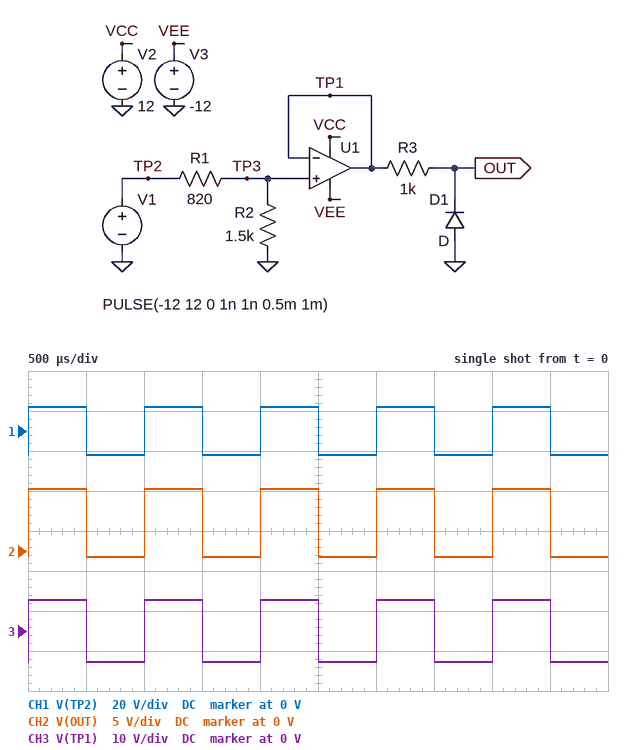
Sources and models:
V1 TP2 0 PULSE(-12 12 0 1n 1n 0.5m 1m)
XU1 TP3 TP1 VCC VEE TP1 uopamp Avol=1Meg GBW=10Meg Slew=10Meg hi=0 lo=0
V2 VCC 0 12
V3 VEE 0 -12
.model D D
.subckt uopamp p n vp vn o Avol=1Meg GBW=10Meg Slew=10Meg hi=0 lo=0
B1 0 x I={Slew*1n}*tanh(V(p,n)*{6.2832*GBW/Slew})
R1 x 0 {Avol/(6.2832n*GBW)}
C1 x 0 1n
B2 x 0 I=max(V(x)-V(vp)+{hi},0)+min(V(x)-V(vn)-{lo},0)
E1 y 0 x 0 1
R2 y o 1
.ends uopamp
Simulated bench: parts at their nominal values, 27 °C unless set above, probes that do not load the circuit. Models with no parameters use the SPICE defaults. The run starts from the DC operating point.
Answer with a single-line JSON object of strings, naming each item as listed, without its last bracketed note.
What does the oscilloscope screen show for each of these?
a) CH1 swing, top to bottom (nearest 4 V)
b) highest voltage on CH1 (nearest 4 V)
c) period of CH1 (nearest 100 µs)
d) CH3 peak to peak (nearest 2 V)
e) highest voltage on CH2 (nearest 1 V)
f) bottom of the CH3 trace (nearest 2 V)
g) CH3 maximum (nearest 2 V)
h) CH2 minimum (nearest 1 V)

{"CH1 swing, top to bottom": "24 V", "highest voltage on CH1": "12 V", "period of CH1": "1.0 ms", "CH3 peak to peak": "16 V", "highest voltage on CH2": "8 V", "bottom of the CH3 trace": "-8 V", "CH3 maximum": "8 V", "CH2 minimum": "-1 V"}
